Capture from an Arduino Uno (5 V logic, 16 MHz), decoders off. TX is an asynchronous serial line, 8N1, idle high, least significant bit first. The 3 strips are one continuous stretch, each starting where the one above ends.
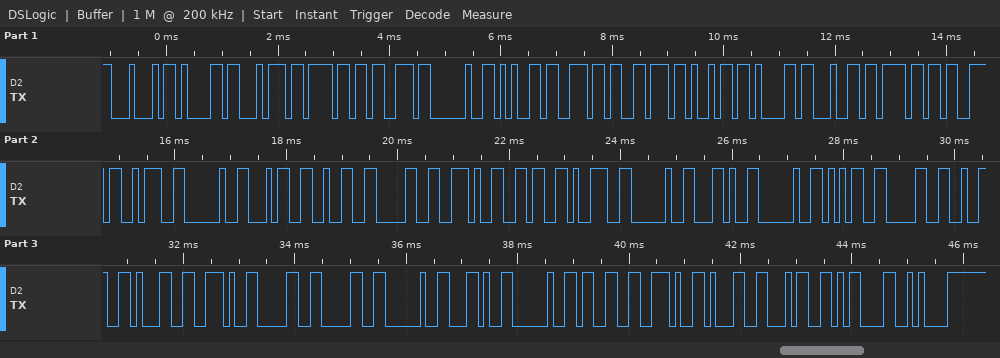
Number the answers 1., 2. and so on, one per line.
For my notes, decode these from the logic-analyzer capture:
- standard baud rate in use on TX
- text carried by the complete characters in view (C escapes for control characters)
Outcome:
1. 9600 baud
2. "Datos enviados: 420.69 , 5021.00 , 3.14\r\n"
